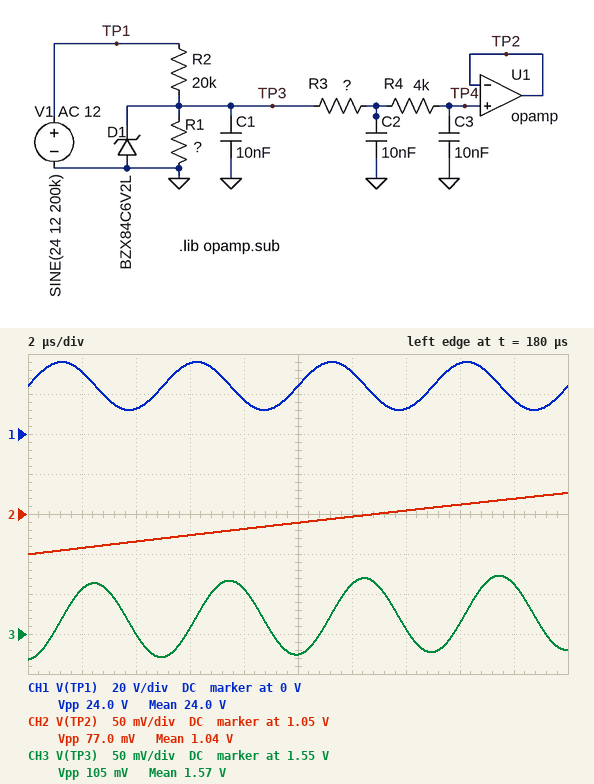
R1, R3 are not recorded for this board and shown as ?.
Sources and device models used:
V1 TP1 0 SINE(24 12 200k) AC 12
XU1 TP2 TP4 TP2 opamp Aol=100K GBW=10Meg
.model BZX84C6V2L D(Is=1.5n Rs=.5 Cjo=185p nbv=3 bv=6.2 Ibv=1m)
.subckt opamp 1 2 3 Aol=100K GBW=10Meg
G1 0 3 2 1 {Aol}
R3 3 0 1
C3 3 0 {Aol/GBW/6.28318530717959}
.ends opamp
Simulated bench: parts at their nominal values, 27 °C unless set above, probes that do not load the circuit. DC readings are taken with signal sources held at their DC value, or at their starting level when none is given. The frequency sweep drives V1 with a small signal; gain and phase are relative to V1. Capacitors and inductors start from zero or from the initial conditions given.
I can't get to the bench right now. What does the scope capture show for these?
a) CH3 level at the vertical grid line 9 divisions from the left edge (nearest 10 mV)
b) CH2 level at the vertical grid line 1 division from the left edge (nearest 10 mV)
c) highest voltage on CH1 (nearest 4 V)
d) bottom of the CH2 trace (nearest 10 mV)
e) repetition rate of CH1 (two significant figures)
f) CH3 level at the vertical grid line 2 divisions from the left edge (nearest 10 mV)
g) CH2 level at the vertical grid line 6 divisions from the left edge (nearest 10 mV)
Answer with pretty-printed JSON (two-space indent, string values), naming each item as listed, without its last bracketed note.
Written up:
{
  "CH3 level at the vertical grid line 9 divisions from the left edge": "1.61 V",
  "CH2 level at the vertical grid line 1 division from the left edge": "1.01 V",
  "highest voltage on CH1": "36 V",
  "bottom of the CH2 trace": "1.00 V",
  "repetition rate of CH1": "200 kHz",
  "CH3 level at the vertical grid line 2 divisions from the left edge": "1.55 V",
  "CH2 level at the vertical grid line 6 divisions from the left edge": "1.05 V"
}
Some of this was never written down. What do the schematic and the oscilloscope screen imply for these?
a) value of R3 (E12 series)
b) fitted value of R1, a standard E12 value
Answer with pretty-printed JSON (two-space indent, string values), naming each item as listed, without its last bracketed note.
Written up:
{
  "value of R3": "5.6 kΩ",
  "fitted value of R1, a standard E12 value": "1.5 kΩ"
}
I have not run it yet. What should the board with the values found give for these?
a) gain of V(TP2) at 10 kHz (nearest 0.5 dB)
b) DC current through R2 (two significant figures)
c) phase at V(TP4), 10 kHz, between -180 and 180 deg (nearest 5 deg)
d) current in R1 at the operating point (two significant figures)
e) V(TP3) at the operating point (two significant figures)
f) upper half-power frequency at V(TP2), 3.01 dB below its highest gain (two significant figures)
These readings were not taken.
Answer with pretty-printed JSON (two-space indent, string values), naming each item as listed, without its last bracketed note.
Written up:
{
  "gain of V(TP2) at 10 kHz": "-48.5 dB",
  "DC current through R2": "1.1 mA",
  "phase at V(TP4), 10 kHz, between -180 and 180 deg": "-165 deg",
  "current in R1 at the operating point": "1.1 mA",
  "V(TP3) at the operating point": "1.7 V",
  "upper half-power frequency at V(TP2), 3.01 dB below its highest gain": "950 Hz"
}
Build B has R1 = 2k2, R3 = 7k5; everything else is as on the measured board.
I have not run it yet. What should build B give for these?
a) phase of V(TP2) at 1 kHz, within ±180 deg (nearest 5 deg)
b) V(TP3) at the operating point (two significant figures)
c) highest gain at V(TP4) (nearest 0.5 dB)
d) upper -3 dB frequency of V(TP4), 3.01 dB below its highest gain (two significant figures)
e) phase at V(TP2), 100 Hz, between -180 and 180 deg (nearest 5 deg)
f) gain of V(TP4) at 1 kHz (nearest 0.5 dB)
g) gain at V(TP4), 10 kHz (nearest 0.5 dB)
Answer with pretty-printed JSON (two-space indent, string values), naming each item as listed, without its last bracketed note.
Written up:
{
  "phase of V(TP2) at 1 kHz, within ±180 deg": "-65 deg",
  "V(TP3) at the operating point": "2.4 V",
  "highest gain at V(TP4)": "-20.0 dB",
  "upper -3 dB frequency of V(TP4), 3.01 dB below its highest gain": "730 Hz",
  "phase at V(TP2), 100 Hz, between -180 and 180 deg": "-10 deg",
  "gain of V(TP4) at 1 kHz": "-24.5 dB",
  "gain at V(TP4), 10 kHz": "-49.5 dB"
}
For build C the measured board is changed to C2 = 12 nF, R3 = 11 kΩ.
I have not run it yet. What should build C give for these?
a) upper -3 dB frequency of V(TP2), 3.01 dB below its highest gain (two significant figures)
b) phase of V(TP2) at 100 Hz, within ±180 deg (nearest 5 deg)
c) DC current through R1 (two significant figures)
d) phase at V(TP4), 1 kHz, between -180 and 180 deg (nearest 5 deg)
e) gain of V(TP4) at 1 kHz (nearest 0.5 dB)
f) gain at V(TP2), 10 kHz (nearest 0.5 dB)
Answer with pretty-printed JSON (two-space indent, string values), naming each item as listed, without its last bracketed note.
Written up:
{
  "upper -3 dB frequency of V(TP2), 3.01 dB below its highest gain": "540 Hz",
  "phase of V(TP2) at 100 Hz, within ±180 deg": "-10 deg",
  "DC current through R1": "1.1 mA",
  "phase at V(TP4), 1 kHz, between -180 and 180 deg": "-75 deg",
  "gain of V(TP4) at 1 kHz": "-29.5 dB",
  "gain at V(TP2), 10 kHz": "-55.0 dB"
}
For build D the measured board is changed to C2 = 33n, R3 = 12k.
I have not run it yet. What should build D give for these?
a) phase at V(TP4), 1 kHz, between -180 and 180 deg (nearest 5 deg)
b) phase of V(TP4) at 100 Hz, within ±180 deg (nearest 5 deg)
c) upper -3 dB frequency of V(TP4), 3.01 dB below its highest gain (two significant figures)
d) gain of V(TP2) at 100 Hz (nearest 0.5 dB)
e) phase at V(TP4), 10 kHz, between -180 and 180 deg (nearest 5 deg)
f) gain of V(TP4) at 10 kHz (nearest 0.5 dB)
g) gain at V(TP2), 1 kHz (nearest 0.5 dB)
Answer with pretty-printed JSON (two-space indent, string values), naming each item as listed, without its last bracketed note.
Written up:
{
  "phase at V(TP4), 1 kHz, between -180 and 180 deg": "-90 deg",
  "phase of V(TP4) at 100 Hz, within ±180 deg": "-20 deg",
  "upper -3 dB frequency of V(TP4), 3.01 dB below its highest gain": "270 Hz",
  "gain of V(TP2) at 100 Hz": "-23.5 dB",
  "phase at V(TP4), 10 kHz, between -180 and 180 deg": "170 deg",
  "gain of V(TP4) at 10 kHz": "-63.0 dB",
  "gain at V(TP2), 1 kHz": "-35.0 dB"
}
